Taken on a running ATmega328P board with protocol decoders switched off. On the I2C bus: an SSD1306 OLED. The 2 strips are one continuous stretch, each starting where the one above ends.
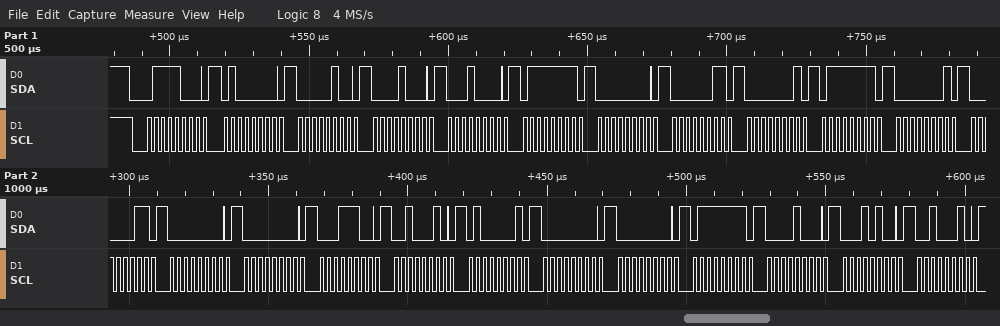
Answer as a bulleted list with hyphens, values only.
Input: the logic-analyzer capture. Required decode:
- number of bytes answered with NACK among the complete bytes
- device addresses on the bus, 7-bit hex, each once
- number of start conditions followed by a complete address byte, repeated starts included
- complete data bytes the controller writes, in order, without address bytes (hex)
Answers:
- 0
- 0x3C
- 1
- 40 04 08 10 7F 00 03 01 7F 01 03 00 00 1C 22 41 00 00 7F 08 14 22
